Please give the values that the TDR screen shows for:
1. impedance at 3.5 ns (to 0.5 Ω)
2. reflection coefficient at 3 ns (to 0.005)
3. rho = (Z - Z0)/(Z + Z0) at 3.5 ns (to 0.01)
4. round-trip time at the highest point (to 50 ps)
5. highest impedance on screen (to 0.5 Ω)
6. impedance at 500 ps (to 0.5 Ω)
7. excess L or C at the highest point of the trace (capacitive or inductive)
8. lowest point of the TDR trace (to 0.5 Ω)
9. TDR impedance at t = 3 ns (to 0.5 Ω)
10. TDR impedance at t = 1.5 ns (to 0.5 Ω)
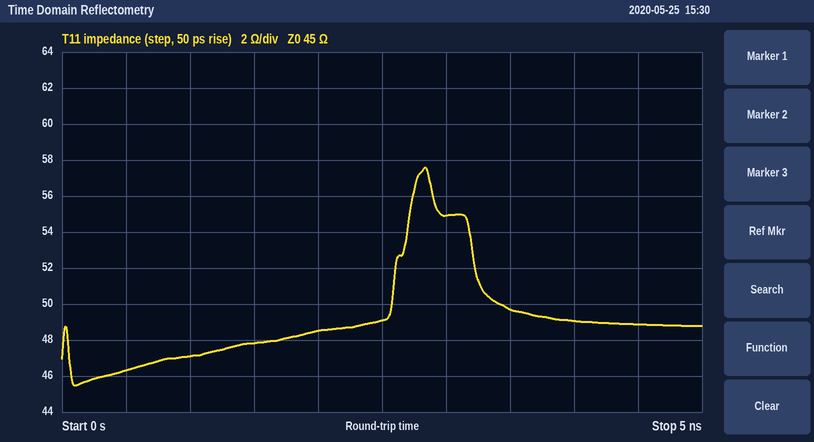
49.5 Ω
+0.100
+0.05
2.85 ns
57.5 Ω
46.5 Ω
inductive
45.5 Ω
55.0 Ω
48.0 Ω
